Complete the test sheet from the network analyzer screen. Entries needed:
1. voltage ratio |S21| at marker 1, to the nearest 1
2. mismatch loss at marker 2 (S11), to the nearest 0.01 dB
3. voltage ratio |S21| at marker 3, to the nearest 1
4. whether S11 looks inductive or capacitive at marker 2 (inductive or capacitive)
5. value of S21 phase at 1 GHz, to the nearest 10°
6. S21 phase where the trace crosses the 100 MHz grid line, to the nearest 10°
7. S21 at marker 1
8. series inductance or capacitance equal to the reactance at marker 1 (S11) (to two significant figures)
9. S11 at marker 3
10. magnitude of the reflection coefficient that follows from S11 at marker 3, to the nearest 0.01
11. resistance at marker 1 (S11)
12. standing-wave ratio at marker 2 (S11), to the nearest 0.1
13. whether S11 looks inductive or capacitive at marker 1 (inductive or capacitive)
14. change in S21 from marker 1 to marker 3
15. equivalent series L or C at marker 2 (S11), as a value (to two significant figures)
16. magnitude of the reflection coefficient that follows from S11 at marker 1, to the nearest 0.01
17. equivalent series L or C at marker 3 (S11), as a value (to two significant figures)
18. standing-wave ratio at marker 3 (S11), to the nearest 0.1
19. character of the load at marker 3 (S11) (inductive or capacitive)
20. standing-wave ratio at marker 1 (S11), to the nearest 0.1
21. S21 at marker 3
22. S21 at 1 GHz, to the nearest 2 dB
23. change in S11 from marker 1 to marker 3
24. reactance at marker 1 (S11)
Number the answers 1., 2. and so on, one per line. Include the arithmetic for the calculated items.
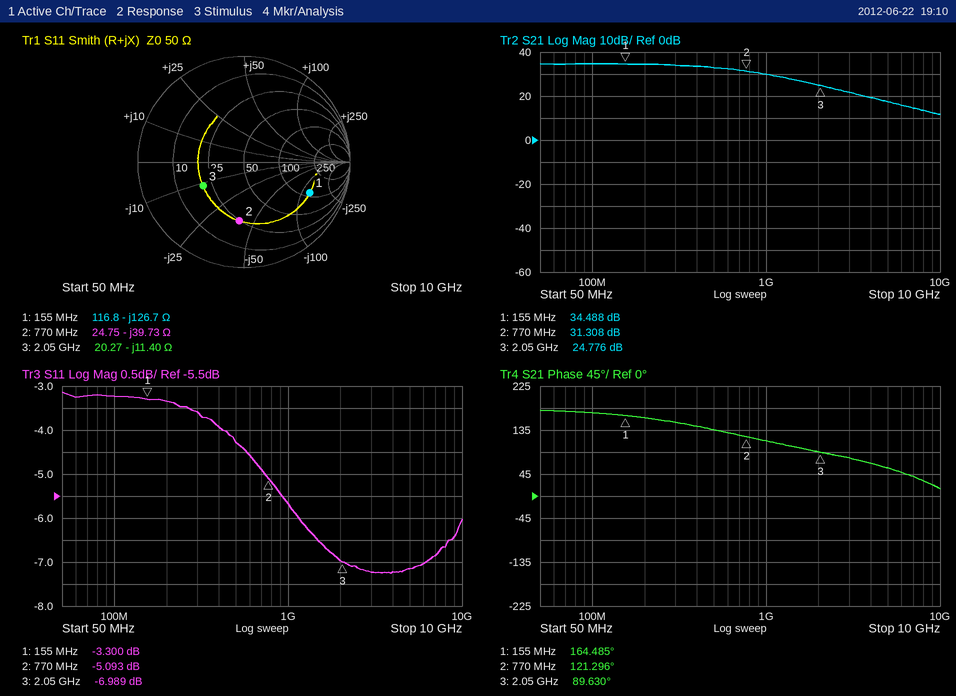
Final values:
1. 10^(34.488/20) ≈ 53
2. −10 log10(1 − 10^(-5.093/10)) ≈ 1.61 dB
3. 10^(24.776/20) ≈ 17
4. capacitive
5. 110°
6. 170°
7. 34.488 dB
8. C = 1/(2π × 155 MHz × 126.7 Ω) ≈ 8.1 pF
9. -6.989 dB
10. 10^(-6.989/20) ≈ 0.45
11. 116.8 Ω
12. 3.5
13. capacitive
14. 24.776 − (34.488) = -9.712 dB
15. C = 1/(2π × 770 MHz × 39.73 Ω) ≈ 5.2 pF
16. 10^(-3.3/20) ≈ 0.68
17. C = 1/(2π × 2.05 GHz × 11.4 Ω) ≈ 6.8 pF
18. 2.6
19. capacitive
20. 5.3
21. 24.776 dB
22. 30 dB
23. -6.989 − (-3.3) = -3.689 dB
24. -126.7 Ω
